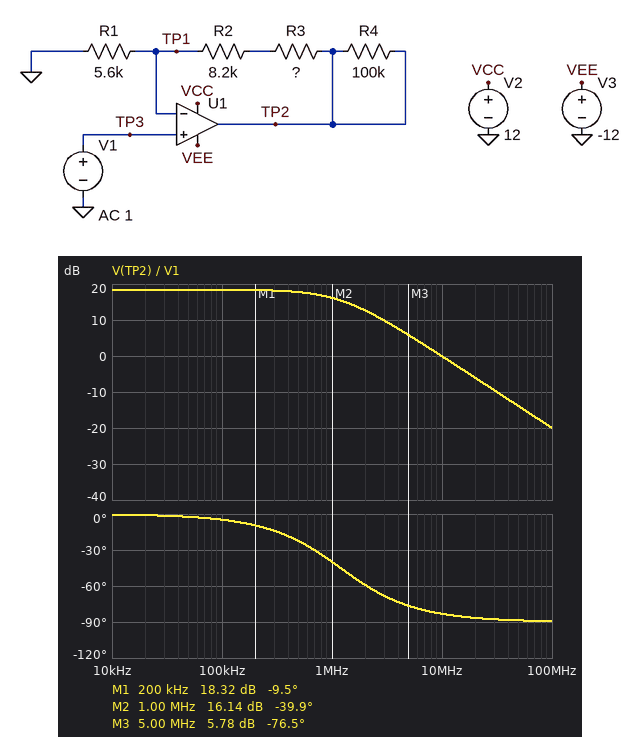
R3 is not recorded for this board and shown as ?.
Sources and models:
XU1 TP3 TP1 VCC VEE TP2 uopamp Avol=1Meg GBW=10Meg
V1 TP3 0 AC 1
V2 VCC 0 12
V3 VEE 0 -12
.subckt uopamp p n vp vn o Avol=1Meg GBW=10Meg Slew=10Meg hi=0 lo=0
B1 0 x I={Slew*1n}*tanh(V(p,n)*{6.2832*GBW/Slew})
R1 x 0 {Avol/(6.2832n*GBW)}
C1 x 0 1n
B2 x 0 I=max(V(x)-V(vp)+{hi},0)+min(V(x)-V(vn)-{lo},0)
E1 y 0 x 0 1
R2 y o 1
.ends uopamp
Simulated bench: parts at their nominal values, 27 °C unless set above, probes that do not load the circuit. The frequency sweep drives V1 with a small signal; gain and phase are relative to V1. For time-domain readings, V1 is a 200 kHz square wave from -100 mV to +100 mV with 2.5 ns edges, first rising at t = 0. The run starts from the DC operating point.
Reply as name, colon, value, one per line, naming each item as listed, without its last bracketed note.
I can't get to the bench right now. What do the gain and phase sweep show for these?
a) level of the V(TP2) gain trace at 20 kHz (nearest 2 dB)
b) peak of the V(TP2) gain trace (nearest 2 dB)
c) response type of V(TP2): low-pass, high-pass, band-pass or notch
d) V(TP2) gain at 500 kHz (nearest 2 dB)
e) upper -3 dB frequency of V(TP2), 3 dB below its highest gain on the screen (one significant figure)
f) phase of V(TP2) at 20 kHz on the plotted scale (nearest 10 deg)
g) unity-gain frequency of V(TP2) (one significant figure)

level of the V(TP2) gain trace at 20 kHz: 18 dB
peak of the V(TP2) gain trace: 18 dB
response type of V(TP2): low-pass, high-pass, band-pass or notch: low-pass
V(TP2) gain at 500 kHz: 18 dB
upper -3 dB frequency of V(TP2), 3 dB below its highest gain on the screen: 1 MHz
phase of V(TP2) at 20 kHz on the plotted scale: 0 deg
unity-gain frequency of V(TP2): 10 MHz
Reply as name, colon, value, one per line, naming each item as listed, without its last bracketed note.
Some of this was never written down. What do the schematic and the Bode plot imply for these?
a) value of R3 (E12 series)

value of R3: 33 kΩ
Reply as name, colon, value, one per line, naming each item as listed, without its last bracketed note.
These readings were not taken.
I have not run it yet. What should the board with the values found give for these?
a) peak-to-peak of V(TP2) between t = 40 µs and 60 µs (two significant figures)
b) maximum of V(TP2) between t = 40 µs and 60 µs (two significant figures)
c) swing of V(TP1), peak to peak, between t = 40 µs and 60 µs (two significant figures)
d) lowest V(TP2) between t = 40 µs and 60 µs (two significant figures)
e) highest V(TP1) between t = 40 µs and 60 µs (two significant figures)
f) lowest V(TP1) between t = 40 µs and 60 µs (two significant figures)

peak-to-peak of V(TP2) between t = 40 µs and 60 µs: 1.7 V
maximum of V(TP2) between t = 40 µs and 60 µs: 840 mV
swing of V(TP1), peak to peak, between t = 40 µs and 60 µs: 200 mV
lowest V(TP2) between t = 40 µs and 60 µs: -840 mV
highest V(TP1) between t = 40 µs and 60 µs: 100 mV
lowest V(TP1) between t = 40 µs and 60 µs: -100 mV
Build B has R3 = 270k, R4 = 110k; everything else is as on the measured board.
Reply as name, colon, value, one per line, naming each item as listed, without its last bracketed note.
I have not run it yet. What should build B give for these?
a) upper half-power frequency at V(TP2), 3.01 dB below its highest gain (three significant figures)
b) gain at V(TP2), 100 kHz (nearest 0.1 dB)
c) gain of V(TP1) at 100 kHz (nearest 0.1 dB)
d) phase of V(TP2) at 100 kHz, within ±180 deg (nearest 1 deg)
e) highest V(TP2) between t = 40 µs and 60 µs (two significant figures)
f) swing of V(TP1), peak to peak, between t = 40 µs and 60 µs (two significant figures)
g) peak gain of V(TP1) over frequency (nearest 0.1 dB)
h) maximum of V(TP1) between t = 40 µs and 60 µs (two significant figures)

upper half-power frequency at V(TP2), 3.01 dB below its highest gain: 197 kHz
gain at V(TP2), 100 kHz: 33.1 dB
gain of V(TP1) at 100 kHz: -1.0 dB
phase of V(TP2) at 100 kHz, within ±180 deg: -27 deg
highest V(TP2) between t = 40 µs and 60 µs: 4.5 V
swing of V(TP1), peak to peak, between t = 40 µs and 60 µs: 180 mV
peak gain of V(TP1) over frequency: 0 dB
maximum of V(TP1) between t = 40 µs and 60 µs: 89 mV
